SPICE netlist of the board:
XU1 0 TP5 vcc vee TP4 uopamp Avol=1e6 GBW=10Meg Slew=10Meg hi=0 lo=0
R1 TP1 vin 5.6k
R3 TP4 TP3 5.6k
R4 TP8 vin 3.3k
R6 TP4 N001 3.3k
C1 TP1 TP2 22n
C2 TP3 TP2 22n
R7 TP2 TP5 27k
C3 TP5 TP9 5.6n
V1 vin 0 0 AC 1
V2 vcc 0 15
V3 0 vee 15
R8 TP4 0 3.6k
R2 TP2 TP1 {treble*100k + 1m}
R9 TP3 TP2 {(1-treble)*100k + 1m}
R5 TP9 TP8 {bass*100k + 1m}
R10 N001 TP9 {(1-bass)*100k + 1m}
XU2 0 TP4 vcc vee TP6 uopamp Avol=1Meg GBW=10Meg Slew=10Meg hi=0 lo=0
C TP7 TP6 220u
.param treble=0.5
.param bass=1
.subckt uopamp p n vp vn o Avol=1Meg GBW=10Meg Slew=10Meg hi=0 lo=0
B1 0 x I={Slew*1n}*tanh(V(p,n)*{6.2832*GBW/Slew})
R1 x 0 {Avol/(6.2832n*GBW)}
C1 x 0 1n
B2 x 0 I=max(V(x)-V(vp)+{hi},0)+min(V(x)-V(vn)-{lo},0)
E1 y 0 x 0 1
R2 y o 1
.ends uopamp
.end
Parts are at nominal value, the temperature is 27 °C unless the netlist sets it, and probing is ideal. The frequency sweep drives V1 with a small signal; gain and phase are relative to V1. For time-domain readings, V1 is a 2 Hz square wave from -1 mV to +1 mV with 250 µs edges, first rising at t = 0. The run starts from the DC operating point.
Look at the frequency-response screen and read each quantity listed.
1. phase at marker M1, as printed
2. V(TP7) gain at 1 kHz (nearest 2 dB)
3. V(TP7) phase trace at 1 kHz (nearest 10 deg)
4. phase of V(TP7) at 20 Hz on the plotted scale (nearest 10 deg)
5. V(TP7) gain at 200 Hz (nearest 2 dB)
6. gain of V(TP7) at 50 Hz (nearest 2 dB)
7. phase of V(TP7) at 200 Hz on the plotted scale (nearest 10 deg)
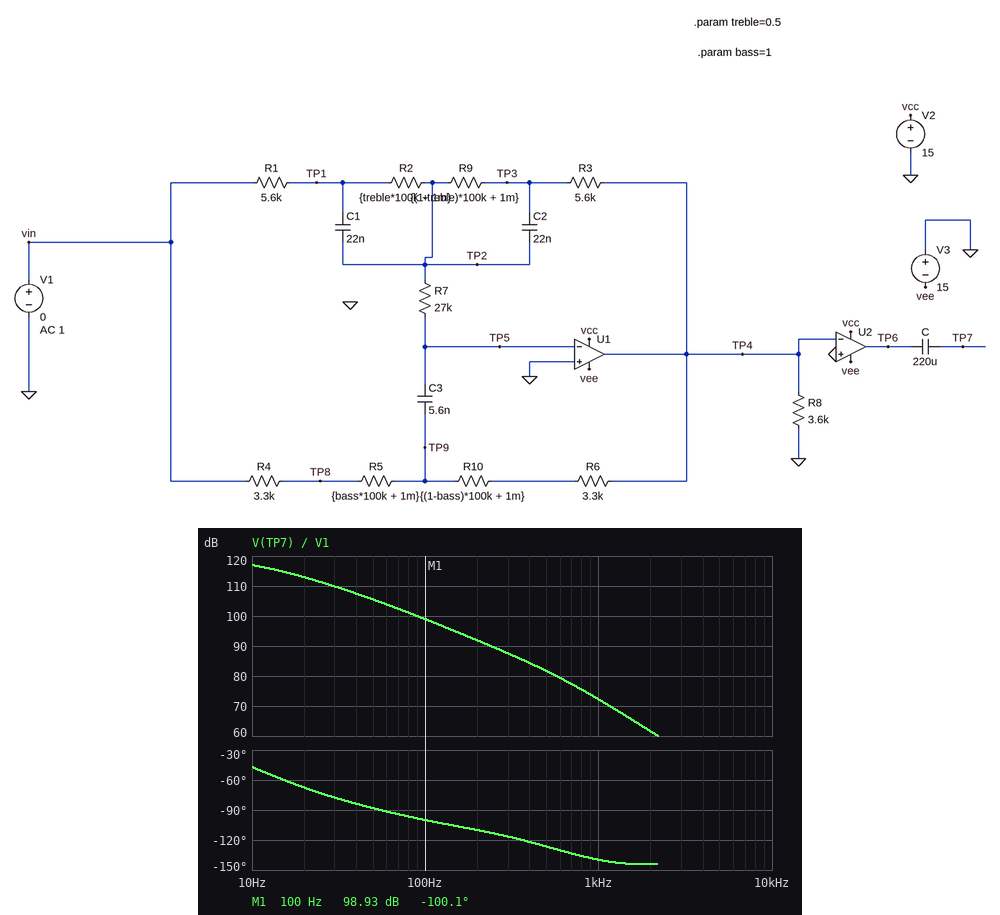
-100.1 deg
72 dB
-140 deg
-70 deg
92 dB
106 dB
-110 deg
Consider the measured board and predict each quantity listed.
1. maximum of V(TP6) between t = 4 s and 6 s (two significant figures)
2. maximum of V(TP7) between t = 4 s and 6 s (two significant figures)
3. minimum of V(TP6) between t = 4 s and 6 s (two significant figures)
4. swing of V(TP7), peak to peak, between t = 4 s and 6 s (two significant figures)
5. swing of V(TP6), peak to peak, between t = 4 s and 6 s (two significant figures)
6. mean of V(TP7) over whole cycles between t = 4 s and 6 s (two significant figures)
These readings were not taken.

15 V
30 V
-15 V
30 V
30 V
15 V
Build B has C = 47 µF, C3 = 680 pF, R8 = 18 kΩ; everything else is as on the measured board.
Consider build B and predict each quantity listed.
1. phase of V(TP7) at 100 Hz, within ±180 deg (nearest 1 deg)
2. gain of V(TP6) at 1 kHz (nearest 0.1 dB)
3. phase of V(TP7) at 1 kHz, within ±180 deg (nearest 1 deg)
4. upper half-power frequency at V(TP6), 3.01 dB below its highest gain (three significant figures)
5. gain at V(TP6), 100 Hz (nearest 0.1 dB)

-86 deg
79.5 dB
-103 deg
10.0 Hz
99.9 dB
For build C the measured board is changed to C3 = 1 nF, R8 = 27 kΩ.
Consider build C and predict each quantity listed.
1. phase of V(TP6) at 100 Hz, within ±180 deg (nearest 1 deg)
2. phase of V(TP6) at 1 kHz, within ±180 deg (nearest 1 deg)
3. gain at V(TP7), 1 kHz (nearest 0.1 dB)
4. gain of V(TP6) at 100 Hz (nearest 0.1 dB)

-87 deg
-108 deg
79.1 dB
99.8 dB
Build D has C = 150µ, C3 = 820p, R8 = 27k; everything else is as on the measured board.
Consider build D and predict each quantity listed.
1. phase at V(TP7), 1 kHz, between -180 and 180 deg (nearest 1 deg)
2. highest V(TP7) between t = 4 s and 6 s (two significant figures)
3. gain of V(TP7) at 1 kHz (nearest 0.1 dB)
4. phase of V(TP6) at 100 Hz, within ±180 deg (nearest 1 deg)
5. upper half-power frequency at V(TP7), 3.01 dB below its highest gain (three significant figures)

-105 deg
30 V
79.3 dB
-87 deg
10.0 Hz
